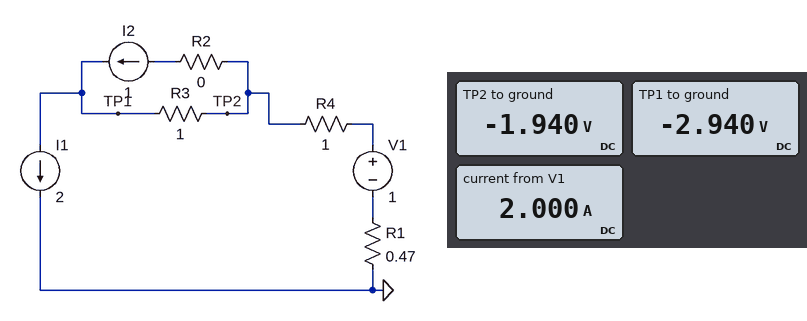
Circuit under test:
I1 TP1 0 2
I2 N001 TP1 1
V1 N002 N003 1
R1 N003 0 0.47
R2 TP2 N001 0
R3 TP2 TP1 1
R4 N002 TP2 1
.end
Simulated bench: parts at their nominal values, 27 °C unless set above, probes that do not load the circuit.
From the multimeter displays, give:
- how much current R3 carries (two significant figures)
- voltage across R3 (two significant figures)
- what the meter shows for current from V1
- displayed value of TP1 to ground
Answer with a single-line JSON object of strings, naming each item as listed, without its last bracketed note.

{"how much current R3 carries": "1.0 A", "voltage across R3": "1.0 V", "what the meter shows for current from V1": "2.000 A", "displayed value of TP1 to ground": "-2.940 V"}
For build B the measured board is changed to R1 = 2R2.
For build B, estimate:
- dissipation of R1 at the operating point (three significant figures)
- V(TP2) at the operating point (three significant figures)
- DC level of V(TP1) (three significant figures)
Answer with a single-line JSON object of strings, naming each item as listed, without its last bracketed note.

{"dissipation of R1 at the operating point": "8.80 W", "V(TP2) at the operating point": "-5.40 V", "DC level of V(TP1)": "-6.40 V"}
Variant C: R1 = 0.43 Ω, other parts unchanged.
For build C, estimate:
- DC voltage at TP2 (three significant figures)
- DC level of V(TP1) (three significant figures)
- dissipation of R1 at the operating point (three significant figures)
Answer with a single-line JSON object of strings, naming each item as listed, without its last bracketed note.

{"DC voltage at TP2": "-1.86 V", "DC level of V(TP1)": "-2.86 V", "dissipation of R1 at the operating point": "1.72 W"}
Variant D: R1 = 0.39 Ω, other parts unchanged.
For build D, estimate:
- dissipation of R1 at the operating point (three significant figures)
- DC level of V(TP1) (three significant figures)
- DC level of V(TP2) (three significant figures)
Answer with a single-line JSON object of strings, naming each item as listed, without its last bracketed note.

{"dissipation of R1 at the operating point": "1.56 W", "DC level of V(TP1)": "-2.78 V", "DC level of V(TP2)": "-1.78 V"}
